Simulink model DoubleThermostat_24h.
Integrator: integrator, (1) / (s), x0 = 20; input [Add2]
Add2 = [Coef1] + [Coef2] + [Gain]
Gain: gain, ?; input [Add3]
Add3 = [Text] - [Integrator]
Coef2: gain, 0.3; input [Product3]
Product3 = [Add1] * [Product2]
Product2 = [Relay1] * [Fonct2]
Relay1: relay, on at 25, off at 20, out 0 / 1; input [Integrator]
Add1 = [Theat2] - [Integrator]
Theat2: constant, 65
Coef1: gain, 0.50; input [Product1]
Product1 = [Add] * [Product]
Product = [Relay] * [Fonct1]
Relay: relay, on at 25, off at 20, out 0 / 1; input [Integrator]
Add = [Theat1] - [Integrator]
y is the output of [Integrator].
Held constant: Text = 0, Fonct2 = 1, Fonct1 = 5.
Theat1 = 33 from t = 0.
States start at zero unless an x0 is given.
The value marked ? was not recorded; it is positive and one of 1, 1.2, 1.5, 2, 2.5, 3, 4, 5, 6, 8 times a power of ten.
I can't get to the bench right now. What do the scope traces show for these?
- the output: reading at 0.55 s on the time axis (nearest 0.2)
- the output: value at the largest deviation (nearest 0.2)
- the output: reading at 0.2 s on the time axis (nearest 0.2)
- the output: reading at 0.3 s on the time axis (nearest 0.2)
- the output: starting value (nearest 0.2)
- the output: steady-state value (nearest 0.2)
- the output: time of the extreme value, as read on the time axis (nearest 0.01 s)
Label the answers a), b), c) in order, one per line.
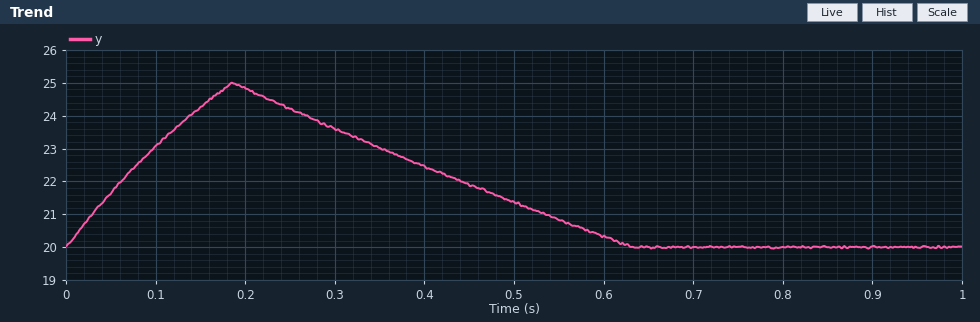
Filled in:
a) 20.8
b) 25.0
c) 24.8
d) 23.6
e) 20.0
f) 20.0
g) 0.19 s
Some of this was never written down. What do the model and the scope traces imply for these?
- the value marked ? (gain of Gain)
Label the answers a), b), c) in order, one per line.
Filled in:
a) 0.5
